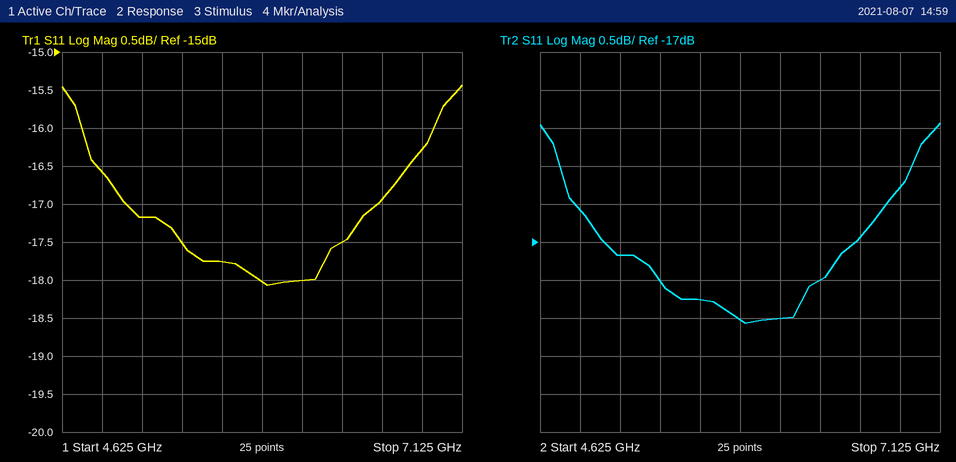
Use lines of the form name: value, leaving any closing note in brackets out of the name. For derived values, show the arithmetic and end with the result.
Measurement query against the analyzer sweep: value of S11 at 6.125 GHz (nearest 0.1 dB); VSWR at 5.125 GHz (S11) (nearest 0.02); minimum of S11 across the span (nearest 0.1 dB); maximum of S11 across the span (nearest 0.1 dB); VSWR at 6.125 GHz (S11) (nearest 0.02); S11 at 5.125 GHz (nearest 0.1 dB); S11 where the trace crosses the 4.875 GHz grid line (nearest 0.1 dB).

value of S11 at 6.125 GHz: -18.0 dB
VSWR at 5.125 GHz (S11): |Γ| = 10^(-17.2/20) = 0.1380; VSWR = (1 + 0.1380)/(1 − 0.1380) ≈ 1.32
minimum of S11 across the span: -18.1 dB
maximum of S11 across the span: -15.4 dB
VSWR at 6.125 GHz (S11): |Γ| = 10^(-18/20) = 0.1259; VSWR = (1 + 0.1259)/(1 − 0.1259) ≈ 1.29, so 1.28 to the nearest 0.02
S11 at 5.125 GHz: -17.2 dB
S11 where the trace crosses the 4.875 GHz grid line: -16.6 dB
